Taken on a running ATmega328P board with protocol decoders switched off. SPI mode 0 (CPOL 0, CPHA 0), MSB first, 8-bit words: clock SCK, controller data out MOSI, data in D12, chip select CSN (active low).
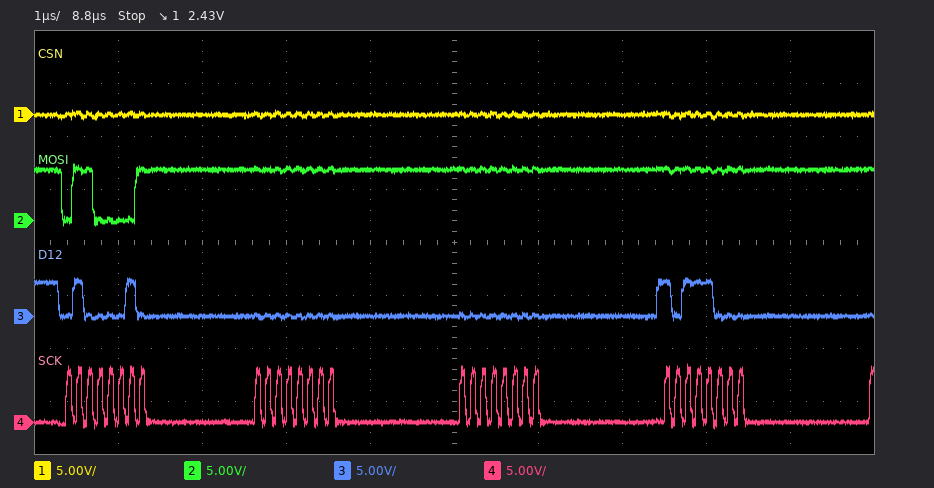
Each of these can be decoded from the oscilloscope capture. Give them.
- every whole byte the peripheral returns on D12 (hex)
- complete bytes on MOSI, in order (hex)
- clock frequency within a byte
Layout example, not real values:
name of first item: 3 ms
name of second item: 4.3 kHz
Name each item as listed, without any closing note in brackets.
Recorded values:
every whole byte the peripheral returns on D12: 42 00 00 B8
complete bytes on MOSI, in order: 61 FF FF FF
clock frequency within a byte: 8 MHz
